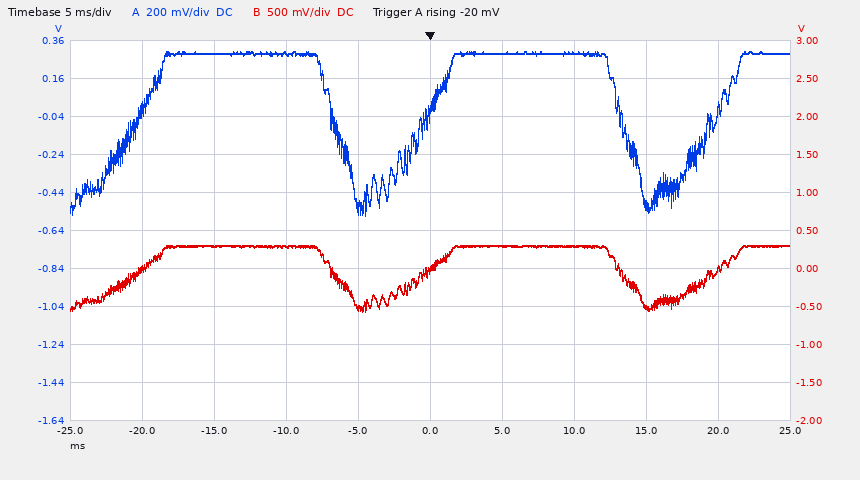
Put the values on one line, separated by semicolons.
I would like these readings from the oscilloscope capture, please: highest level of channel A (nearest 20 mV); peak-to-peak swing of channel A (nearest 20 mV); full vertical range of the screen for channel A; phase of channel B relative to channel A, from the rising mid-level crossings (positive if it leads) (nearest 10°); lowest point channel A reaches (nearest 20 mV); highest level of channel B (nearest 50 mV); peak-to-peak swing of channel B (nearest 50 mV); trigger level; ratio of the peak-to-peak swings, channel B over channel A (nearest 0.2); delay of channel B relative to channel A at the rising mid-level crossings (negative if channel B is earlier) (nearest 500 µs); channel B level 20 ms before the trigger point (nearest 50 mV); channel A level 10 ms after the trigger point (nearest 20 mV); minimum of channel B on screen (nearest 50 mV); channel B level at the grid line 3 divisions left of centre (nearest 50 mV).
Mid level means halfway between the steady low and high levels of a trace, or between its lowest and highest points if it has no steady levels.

300 mV; 860 mV; 2 V; 0°; -560 mV; 300 mV; 850 mV; -20 mV; 1.0; 0.0 ms; 0 mV; 300 mV; -550 mV; 300 mV
